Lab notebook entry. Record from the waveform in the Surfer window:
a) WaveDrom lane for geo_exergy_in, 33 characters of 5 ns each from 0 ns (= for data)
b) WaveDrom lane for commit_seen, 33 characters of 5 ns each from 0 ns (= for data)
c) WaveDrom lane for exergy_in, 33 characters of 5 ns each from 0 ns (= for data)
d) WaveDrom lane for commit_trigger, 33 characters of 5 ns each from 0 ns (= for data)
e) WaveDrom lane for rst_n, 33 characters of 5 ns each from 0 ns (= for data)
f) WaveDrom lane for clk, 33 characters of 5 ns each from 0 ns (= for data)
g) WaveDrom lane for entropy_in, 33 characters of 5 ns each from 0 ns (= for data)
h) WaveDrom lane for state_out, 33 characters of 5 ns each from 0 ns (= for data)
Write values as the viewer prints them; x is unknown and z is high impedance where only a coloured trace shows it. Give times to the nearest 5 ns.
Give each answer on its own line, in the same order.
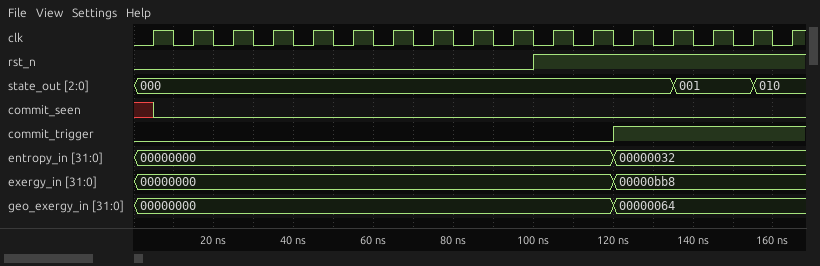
{name: 'geo_exergy_in', wave: '=.......................=........', data: '00000000 00000064'}
{name: 'commit_seen', wave: 'x0...............................'}
{name: 'exergy_in', wave: '=.......................=........', data: '00000000 00000bb8'}
{name: 'commit_trigger', wave: '0.......................1........'}
{name: 'rst_n', wave: '0...................1............'}
{name: 'clk', wave: '010101010101010101010101010101010'}
{name: 'entropy_in', wave: '=.......................=........', data: '00000000 00000032'}
{name: 'state_out', wave: '=..........................=...=.', data: '000 001 010'}
